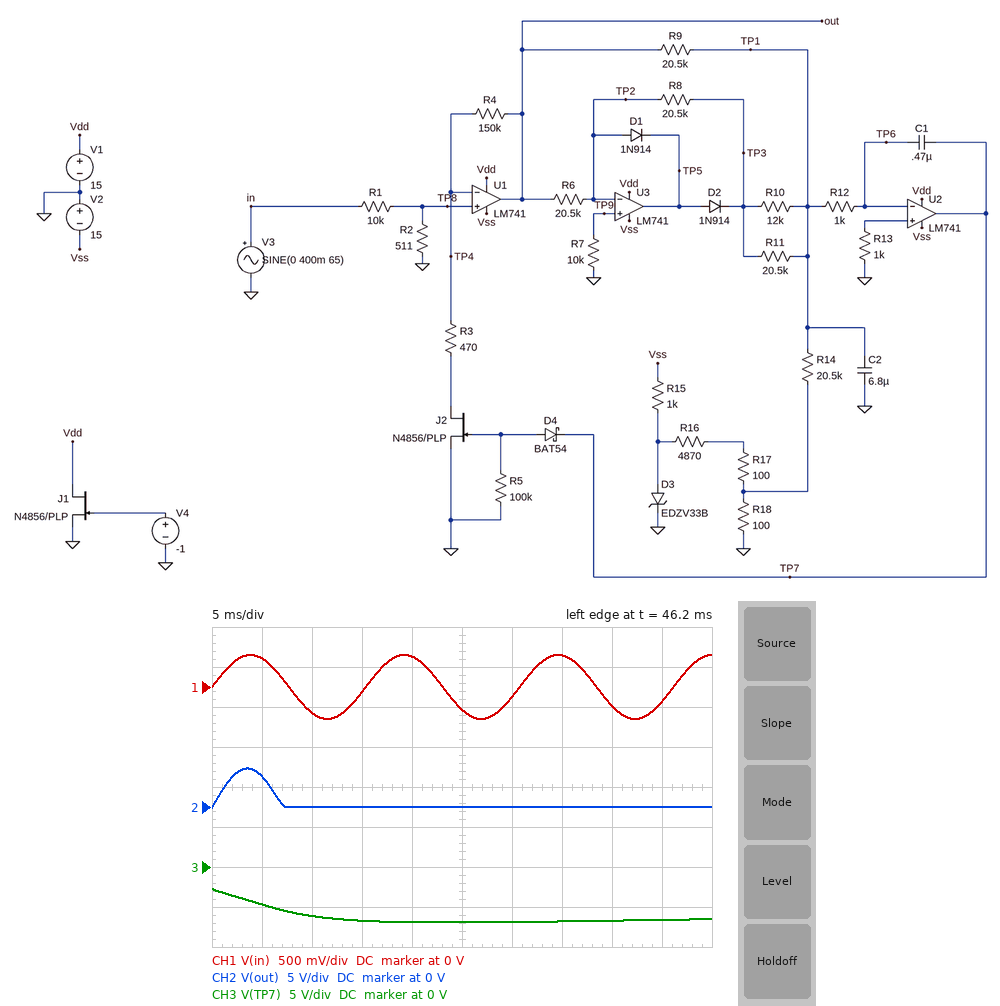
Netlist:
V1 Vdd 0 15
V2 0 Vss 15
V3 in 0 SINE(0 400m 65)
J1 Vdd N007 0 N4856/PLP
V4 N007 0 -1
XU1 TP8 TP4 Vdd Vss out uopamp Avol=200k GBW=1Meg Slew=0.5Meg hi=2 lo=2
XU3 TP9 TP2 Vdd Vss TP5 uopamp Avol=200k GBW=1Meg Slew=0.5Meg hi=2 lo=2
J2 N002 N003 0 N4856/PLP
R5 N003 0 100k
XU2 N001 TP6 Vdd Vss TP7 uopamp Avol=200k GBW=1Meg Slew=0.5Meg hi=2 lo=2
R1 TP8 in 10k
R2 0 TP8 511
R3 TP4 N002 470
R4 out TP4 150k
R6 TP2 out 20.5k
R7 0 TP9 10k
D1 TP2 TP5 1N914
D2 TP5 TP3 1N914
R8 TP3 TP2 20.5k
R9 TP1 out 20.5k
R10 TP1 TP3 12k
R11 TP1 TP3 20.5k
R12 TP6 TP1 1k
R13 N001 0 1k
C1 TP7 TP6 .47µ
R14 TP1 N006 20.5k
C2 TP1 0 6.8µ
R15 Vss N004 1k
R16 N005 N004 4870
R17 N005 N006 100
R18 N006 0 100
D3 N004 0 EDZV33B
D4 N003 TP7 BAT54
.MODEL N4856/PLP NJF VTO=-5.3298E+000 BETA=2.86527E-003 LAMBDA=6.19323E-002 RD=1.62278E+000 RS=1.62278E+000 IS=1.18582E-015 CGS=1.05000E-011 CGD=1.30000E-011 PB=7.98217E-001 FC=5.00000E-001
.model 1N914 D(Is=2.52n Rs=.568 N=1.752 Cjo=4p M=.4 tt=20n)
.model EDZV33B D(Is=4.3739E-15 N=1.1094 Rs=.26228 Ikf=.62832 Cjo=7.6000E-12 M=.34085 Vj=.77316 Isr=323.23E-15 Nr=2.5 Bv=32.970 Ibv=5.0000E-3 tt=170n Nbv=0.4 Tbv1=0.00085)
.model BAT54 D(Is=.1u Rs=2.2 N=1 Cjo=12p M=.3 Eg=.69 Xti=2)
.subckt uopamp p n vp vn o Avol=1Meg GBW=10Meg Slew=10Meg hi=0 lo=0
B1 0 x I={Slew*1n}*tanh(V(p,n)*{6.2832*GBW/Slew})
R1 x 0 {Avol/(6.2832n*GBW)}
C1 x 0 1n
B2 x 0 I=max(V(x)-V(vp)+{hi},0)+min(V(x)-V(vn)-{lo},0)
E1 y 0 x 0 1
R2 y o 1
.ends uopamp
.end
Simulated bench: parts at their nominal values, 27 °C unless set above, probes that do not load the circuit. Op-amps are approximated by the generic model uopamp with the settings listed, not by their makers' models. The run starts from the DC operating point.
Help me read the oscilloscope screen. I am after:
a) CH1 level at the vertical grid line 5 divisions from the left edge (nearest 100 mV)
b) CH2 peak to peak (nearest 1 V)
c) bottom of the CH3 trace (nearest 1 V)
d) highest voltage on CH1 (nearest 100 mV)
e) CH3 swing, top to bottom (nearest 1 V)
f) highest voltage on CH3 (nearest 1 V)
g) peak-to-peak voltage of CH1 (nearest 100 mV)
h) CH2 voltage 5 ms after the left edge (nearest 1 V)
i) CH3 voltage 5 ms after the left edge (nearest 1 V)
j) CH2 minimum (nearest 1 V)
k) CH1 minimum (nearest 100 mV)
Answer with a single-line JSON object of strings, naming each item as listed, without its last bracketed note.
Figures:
{"CH1 level at the vertical grid line 5 divisions from the left edge": "-300 mV", "CH2 peak to peak": "5 V", "bottom of the CH3 trace": "-7 V", "highest voltage on CH1": "400 mV", "CH3 swing, top to bottom": "4 V", "highest voltage on CH3": "-3 V", "peak-to-peak voltage of CH1": "800 mV", "CH2 voltage 5 ms after the left edge": "4 V", "CH3 voltage 5 ms after the left edge": "-5 V", "CH2 minimum": "0 V", "CH1 minimum": "-400 mV"}
